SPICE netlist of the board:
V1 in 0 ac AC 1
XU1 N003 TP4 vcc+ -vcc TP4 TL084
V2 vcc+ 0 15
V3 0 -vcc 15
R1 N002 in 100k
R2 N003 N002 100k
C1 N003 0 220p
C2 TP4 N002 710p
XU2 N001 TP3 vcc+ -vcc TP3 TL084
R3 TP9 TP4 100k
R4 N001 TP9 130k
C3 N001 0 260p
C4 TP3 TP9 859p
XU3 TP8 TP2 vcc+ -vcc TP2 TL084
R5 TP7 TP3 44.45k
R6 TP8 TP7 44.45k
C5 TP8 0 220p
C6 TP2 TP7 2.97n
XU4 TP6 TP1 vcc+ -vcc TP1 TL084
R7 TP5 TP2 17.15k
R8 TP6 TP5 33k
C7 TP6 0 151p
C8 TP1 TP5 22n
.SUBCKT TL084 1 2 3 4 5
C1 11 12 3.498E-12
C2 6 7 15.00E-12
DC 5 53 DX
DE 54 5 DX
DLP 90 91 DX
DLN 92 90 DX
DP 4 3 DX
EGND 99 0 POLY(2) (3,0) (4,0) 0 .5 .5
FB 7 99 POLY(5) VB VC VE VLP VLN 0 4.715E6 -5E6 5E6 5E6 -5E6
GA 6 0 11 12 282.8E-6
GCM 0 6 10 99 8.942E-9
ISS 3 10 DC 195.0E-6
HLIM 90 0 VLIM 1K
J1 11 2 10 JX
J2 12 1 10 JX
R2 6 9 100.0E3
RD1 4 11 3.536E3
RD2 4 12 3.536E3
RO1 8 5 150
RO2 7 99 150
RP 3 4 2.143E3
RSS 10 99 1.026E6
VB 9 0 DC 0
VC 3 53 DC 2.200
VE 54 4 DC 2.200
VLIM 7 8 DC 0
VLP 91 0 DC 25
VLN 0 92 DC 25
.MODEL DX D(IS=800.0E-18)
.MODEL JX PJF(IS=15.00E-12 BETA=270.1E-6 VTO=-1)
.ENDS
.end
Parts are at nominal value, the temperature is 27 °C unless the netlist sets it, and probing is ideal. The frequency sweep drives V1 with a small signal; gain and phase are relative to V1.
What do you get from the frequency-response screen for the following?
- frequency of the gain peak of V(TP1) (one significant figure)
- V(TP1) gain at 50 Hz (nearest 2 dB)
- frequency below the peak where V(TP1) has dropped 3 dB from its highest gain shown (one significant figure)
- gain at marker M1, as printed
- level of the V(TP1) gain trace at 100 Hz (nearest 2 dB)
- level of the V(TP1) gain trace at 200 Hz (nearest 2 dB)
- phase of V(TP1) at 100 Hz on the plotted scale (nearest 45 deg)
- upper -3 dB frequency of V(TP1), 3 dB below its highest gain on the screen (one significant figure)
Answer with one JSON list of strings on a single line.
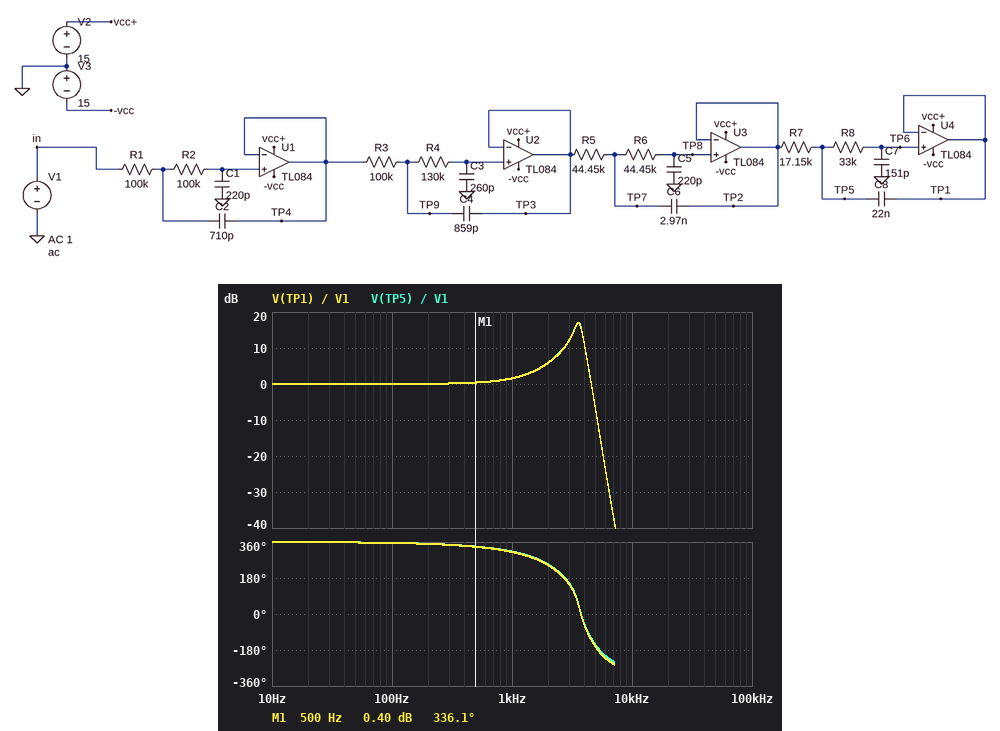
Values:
["4 kHz", "0 dB", "3 kHz", "0.40 dB", "0 dB", "0 dB", "360 deg", "4 kHz"]
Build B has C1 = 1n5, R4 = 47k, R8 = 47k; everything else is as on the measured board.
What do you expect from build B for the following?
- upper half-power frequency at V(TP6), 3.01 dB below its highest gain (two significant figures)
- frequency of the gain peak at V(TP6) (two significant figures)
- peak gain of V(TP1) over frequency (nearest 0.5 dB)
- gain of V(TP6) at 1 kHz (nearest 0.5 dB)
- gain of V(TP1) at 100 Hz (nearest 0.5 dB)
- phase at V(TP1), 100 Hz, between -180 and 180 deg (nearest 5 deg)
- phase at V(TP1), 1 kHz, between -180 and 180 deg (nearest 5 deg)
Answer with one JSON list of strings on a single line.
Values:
["3.3 kHz", "3.0 kHz", "2.5 dB", "-4.5 dB", "0 dB", "-15 deg", "-100 deg"]
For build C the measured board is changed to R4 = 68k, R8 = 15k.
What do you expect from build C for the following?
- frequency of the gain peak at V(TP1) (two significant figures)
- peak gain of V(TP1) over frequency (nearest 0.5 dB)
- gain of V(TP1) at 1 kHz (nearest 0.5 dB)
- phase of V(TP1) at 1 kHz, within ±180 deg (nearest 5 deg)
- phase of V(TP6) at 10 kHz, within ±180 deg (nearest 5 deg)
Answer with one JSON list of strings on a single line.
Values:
["4.3 kHz", "10.5 dB", "1.0 dB", "-40 deg", "80 deg"]
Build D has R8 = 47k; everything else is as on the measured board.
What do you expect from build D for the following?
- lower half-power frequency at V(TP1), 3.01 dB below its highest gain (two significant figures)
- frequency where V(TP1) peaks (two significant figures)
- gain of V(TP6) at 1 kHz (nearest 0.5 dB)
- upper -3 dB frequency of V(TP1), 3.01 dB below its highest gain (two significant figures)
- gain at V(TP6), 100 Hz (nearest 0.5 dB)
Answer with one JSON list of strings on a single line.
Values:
["2.7 kHz", "3.0 kHz", "2.0 dB", "3.3 kHz", "0 dB"]
